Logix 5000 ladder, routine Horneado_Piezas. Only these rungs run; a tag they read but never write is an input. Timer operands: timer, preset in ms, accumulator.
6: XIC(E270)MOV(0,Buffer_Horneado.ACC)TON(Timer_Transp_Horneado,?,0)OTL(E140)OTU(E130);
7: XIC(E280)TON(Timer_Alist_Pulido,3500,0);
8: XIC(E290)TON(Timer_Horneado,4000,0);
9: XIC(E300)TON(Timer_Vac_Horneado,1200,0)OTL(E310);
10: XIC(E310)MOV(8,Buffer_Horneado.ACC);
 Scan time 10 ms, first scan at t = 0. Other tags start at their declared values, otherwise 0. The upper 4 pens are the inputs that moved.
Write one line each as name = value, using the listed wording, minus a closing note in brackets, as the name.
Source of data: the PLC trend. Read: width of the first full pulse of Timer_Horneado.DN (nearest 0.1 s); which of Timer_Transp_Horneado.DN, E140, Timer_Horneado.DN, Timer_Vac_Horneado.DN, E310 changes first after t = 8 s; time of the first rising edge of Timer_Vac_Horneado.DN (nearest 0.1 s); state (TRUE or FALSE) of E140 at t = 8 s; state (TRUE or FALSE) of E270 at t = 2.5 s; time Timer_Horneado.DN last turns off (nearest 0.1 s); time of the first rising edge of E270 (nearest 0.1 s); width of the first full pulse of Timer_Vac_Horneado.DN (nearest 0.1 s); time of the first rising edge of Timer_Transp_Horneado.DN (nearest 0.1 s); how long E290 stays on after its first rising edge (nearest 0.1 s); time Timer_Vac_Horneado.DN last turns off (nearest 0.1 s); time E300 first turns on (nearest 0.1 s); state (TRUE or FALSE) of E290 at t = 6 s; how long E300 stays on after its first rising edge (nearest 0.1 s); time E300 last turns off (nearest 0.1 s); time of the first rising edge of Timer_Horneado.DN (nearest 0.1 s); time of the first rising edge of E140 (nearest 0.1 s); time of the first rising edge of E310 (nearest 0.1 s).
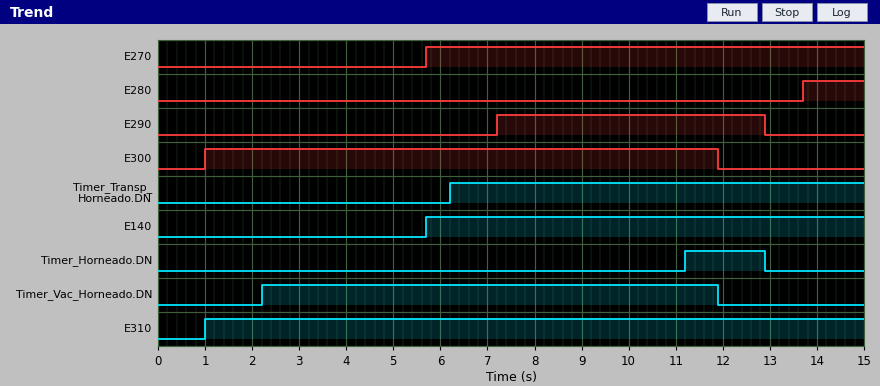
width of the first full pulse of Timer_Horneado.DN = 1.7 s
which of Timer_Transp_Horneado.DN, E140, Timer_Horneado.DN, Timer_Vac_Horneado.DN, E310 changes first after t = 8 s = Timer_Horneado.DN
time of the first rising edge of Timer_Vac_Horneado.DN = 2.2 s
state (TRUE or FALSE) of E140 at t = 8 s = TRUE
state (TRUE or FALSE) of E270 at t = 2.5 s = FALSE
time Timer_Horneado.DN last turns off = 12.9 s
time of the first rising edge of E270 = 5.7 s
width of the first full pulse of Timer_Vac_Horneado.DN = 9.7 s
time of the first rising edge of Timer_Transp_Horneado.DN = 6.2 s
how long E290 stays on after its first rising edge = 5.7 s
time Timer_Vac_Horneado.DN last turns off = 11.9 s
time E300 first turns on = 1.0 s
state (TRUE or FALSE) of E290 at t = 6 s = FALSE
how long E300 stays on after its first rising edge = 10.9 s
time E300 last turns off = 11.9 s
time of the first rising edge of Timer_Horneado.DN = 11.2 s
time of the first rising edge of E140 = 5.7 s
time of the first rising edge of E310 = 1.0 s
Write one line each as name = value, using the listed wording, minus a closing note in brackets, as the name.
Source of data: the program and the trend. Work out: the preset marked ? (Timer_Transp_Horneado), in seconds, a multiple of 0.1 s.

the preset marked ? (Timer_Transp_Horneado), in seconds, a multiple of 0.1 s = 0.5 s
